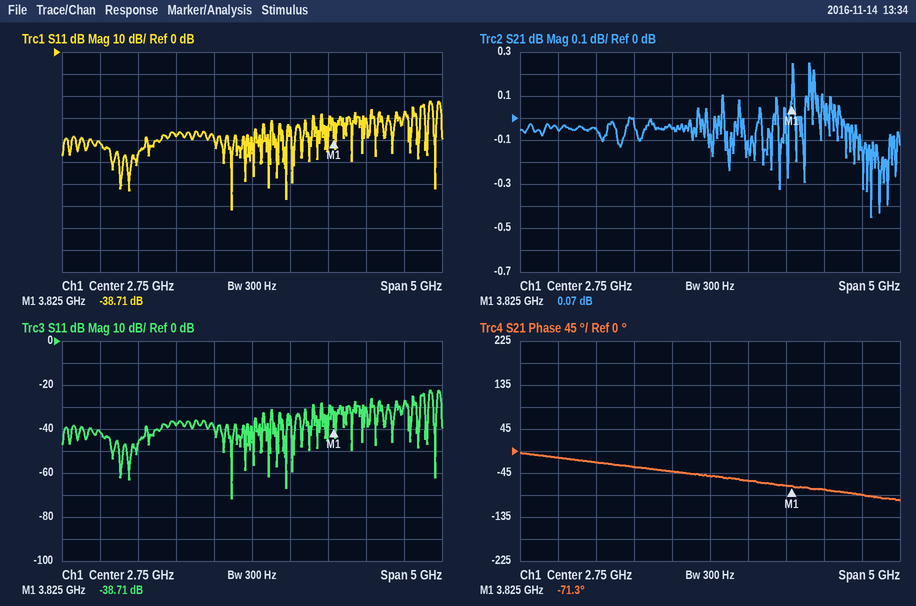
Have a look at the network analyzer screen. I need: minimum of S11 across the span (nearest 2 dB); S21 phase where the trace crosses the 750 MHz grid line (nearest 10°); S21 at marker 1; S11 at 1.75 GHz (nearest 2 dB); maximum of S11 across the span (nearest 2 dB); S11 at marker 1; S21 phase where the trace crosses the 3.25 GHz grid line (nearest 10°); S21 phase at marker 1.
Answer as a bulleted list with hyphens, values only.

- -72 dB
- -10°
- 0.07 dB
- -38 dB
- -22 dB
- -38.71 dB
- -60°
- -71.3°
